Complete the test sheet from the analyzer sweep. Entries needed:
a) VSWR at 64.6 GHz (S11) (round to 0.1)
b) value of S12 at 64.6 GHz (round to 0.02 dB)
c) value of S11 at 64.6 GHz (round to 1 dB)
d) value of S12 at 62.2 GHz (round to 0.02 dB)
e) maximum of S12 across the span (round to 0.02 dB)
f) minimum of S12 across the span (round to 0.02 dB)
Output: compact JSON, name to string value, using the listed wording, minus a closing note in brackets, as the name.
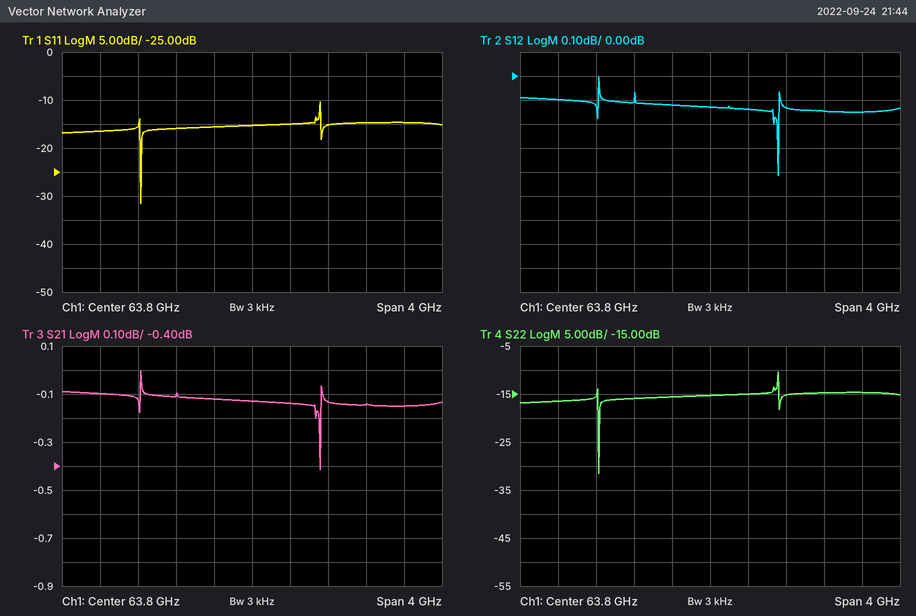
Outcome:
{"VSWR at 64.6 GHz (S11)": "1.4", "value of S12 at 64.6 GHz": "-0.14 dB", "value of S11 at 64.6 GHz": "-15 dB", "value of S12 at 62.2 GHz": "-0.10 dB", "maximum of S12 across the span": "0.00 dB", "minimum of S12 across the span": "-0.42 dB"}
